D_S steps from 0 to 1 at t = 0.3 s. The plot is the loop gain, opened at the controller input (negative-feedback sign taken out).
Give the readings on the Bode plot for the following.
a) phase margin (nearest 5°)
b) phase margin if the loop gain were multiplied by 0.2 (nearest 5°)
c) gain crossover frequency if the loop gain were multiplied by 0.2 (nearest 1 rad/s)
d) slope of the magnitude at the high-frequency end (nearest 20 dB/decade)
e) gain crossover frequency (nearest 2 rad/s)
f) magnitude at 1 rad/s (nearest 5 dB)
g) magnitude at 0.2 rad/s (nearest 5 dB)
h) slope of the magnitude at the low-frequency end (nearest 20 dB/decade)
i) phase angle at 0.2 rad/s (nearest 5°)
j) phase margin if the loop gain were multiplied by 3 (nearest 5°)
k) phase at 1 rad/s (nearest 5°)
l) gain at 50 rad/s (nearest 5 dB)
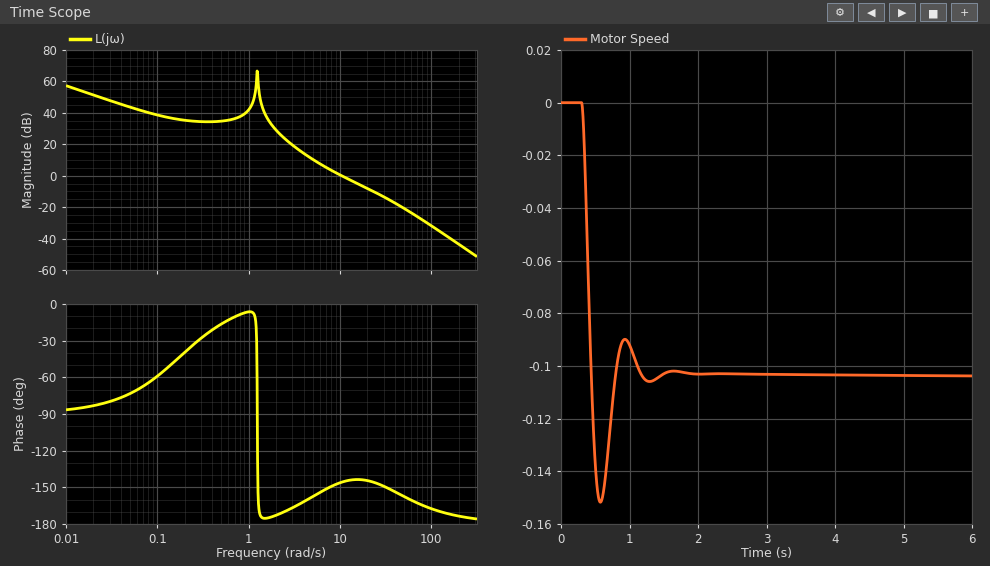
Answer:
35°
20°
4 rad/s
-40 dB/decade
10 rad/s
40 dB
35 dB
-20 dB/decade
-40°
35°
-5°
-20 dB
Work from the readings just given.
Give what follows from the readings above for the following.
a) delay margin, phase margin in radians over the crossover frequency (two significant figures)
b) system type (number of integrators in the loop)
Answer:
0.061 s
1
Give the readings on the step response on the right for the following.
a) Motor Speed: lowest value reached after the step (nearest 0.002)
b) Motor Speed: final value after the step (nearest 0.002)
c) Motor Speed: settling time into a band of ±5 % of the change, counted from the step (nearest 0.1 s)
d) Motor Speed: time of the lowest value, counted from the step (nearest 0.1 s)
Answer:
-0.152
-0.104
0.8 s
0.3 s
